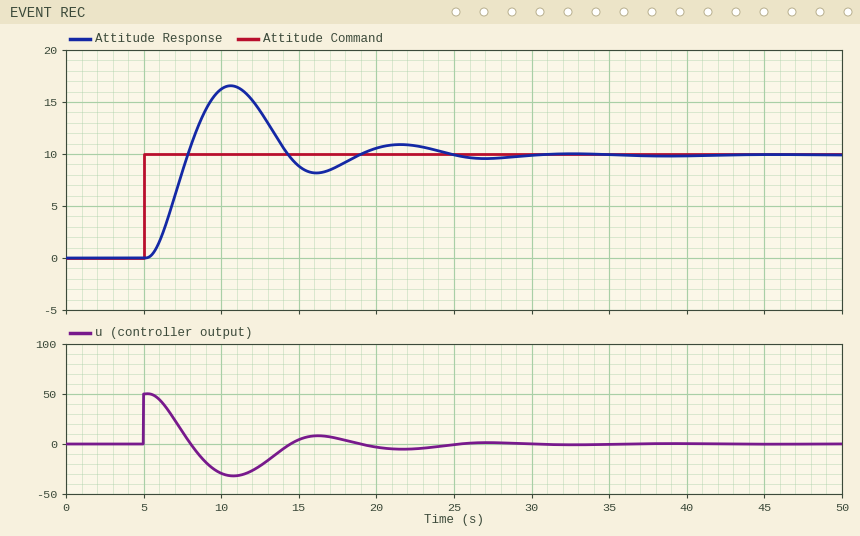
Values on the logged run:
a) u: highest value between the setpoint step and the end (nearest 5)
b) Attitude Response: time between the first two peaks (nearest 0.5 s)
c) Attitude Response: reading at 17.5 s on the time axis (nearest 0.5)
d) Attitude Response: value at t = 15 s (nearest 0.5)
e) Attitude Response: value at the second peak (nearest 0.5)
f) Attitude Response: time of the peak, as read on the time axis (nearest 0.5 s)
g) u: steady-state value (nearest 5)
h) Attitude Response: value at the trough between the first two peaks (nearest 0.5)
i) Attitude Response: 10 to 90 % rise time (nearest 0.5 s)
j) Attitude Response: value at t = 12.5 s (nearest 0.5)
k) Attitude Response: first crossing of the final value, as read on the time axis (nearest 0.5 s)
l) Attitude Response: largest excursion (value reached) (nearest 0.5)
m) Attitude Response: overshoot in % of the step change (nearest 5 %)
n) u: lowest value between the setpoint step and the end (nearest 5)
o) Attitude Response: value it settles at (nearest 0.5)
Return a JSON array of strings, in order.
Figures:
["50", "11.0 s", "9.0", "9.0", "11.0", "10.5 s", "0", "8.0", "2.0 s", "14.0", "8.0 s", "16.5", "65 %", "-30", "10.0"]
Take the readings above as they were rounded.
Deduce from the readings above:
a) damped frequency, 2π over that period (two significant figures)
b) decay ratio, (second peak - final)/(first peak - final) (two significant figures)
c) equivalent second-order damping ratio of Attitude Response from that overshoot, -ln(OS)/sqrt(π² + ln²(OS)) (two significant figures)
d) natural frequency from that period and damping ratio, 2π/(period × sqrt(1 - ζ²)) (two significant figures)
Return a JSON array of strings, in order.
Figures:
["0.57 rad/s", "0.15", "0.14", "0.58 rad/s"]
